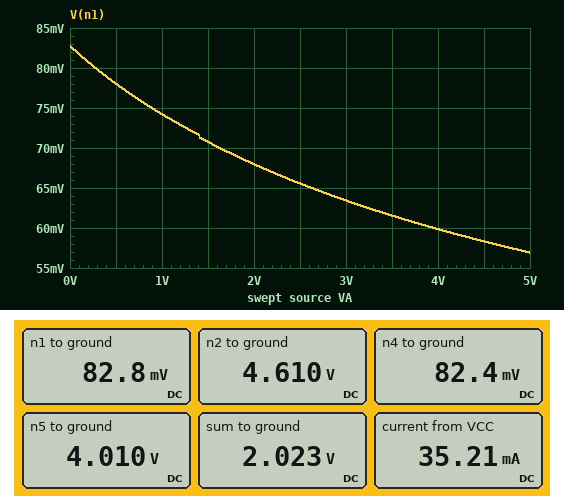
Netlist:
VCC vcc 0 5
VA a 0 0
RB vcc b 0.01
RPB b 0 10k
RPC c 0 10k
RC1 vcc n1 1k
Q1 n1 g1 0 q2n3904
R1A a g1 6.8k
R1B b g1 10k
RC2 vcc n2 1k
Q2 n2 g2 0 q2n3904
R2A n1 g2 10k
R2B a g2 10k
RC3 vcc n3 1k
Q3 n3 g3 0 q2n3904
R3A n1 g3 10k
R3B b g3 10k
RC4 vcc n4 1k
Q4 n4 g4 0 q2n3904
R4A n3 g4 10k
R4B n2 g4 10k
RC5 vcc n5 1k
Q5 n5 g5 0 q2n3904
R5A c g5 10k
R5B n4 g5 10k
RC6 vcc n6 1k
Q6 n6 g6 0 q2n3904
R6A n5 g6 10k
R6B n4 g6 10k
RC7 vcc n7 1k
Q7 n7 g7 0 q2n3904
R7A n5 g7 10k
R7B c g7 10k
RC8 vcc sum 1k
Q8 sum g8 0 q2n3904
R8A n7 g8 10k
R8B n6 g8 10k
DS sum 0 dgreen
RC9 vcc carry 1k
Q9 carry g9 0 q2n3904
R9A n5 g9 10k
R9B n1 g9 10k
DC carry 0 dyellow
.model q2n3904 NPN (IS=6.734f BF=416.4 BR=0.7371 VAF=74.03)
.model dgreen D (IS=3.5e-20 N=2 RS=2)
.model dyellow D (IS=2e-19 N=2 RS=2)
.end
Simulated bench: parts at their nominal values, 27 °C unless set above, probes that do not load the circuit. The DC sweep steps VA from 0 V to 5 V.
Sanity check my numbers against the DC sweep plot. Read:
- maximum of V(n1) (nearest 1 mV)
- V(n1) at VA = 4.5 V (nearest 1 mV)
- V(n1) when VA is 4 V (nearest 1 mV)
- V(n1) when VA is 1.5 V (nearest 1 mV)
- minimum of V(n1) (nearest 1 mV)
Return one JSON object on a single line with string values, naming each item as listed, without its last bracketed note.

{"maximum of V(n1)": "83 mV", "V(n1) at VA = 4.5 V": "58 mV", "V(n1) when VA is 4 V": "60 mV", "V(n1) when VA is 1.5 V": "71 mV", "minimum of V(n1)": "57 mV"}
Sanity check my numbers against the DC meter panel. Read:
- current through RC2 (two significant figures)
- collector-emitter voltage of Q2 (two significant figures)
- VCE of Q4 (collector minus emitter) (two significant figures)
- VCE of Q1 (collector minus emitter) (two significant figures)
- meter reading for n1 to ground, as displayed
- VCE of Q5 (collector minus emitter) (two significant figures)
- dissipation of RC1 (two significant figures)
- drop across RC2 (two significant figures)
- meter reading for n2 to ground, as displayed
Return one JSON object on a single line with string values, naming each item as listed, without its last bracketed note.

{"current through RC2": "390 µA", "collector-emitter voltage of Q2": "4.6 V", "VCE of Q4 (collector minus emitter)": "82 mV", "VCE of Q1 (collector minus emitter)": "83 mV", "meter reading for n1 to ground, as displayed": "82.8 mV", "VCE of Q5 (collector minus emitter)": "4.0 V", "dissipation of RC1": "24 mW", "drop across RC2": "390 mV", "meter reading for n2 to ground, as displayed": "4.610 V"}
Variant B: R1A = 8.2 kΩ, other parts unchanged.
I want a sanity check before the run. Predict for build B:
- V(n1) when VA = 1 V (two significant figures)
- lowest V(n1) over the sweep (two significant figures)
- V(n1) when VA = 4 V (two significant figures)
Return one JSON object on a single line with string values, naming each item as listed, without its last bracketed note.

{"V(n1) when VA = 1 V": "75 mV", "lowest V(n1) over the sweep": "59 mV", "V(n1) when VA = 4 V": "62 mV"}
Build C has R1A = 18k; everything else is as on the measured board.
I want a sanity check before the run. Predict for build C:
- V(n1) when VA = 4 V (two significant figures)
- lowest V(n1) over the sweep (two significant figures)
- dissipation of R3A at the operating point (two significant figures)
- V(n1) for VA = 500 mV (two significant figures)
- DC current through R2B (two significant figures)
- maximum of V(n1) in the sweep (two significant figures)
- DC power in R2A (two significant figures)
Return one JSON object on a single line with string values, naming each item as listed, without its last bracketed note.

{"V(n1) when VA = 4 V": "68 mV", "lowest V(n1) over the sweep": "66 mV", "dissipation of R3A at the operating point": "40 µW", "V(n1) for VA = 500 mV": "77 mV", "DC current through R2B": "3.9 µA", "maximum of V(n1) in the sweep": "78 mV", "DC power in R2A": "150 nW"}
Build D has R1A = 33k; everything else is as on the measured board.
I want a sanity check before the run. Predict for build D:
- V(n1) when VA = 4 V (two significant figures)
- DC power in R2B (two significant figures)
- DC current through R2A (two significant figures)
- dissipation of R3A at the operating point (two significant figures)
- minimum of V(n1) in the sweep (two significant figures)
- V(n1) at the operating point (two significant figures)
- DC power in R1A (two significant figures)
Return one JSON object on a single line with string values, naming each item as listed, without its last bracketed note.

{"V(n1) when VA = 4 V": "71 mV", "DC power in R2B": "150 nW", "DC current through R2A": "3.9 µA", "dissipation of R3A at the operating point": "40 µW", "minimum of V(n1) in the sweep": "70 mV", "V(n1) at the operating point": "77 mV", "DC power in R1A": "15 µW"}
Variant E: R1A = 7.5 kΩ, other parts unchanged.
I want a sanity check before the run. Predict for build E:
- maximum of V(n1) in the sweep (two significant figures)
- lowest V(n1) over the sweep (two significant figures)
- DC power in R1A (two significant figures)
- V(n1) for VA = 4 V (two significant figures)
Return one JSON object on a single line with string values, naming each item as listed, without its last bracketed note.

{"maximum of V(n1) in the sweep": "82 mV", "lowest V(n1) over the sweep": "58 mV", "DC power in R1A": "67 µW", "V(n1) for VA = 4 V": "61 mV"}
